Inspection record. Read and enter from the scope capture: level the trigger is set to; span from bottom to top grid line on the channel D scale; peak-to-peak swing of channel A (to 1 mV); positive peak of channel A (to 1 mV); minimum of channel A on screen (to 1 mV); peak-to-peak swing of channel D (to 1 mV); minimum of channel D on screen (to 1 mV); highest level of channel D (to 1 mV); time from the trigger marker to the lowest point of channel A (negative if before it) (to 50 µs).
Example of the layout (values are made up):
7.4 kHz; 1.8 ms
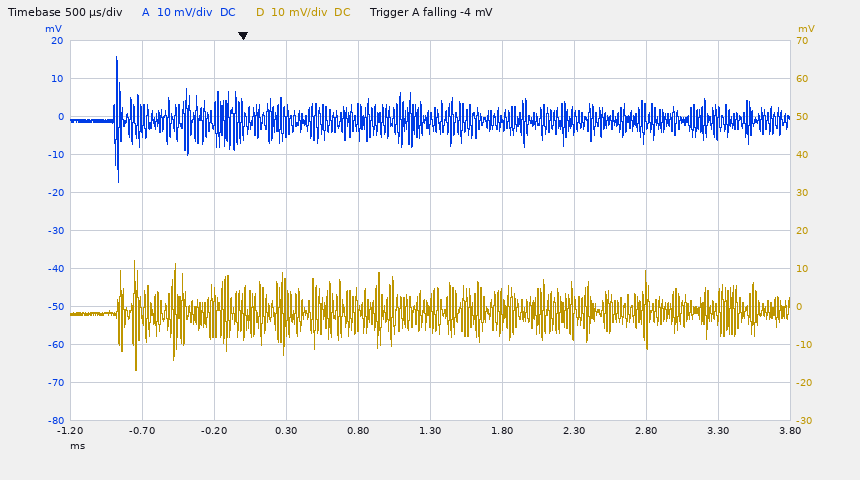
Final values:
-4 mV; 100 mV; 33 mV; 16 mV; -17 mV; 29 mV; -17 mV; 12 mV; -850 µs
